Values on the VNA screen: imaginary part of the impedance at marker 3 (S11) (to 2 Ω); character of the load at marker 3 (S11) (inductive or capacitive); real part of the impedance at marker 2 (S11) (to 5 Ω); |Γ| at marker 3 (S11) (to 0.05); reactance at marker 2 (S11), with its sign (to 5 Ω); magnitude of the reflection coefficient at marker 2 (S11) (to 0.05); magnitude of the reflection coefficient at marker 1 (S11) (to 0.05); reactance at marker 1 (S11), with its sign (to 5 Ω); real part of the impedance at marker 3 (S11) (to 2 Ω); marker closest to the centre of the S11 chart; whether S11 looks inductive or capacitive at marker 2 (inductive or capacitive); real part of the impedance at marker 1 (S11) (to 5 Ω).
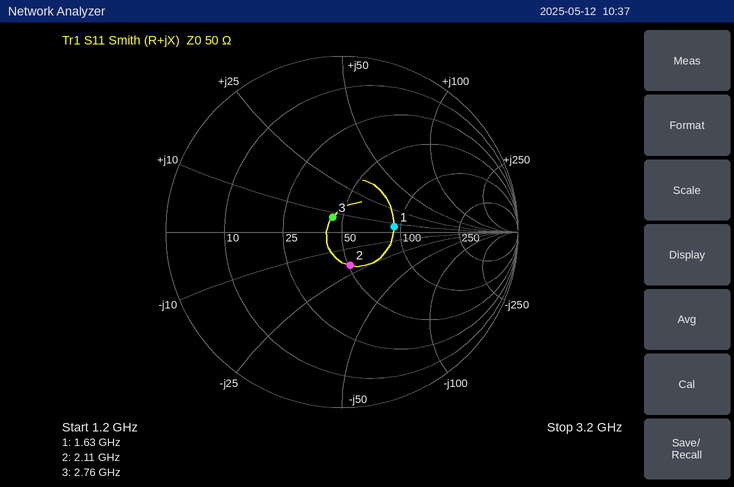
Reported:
+8 Ω
inductive
50 Ω
0.10
-20 Ω
0.20
0.30
+5 Ω
44 Ω
marker 3
capacitive
90 Ω
